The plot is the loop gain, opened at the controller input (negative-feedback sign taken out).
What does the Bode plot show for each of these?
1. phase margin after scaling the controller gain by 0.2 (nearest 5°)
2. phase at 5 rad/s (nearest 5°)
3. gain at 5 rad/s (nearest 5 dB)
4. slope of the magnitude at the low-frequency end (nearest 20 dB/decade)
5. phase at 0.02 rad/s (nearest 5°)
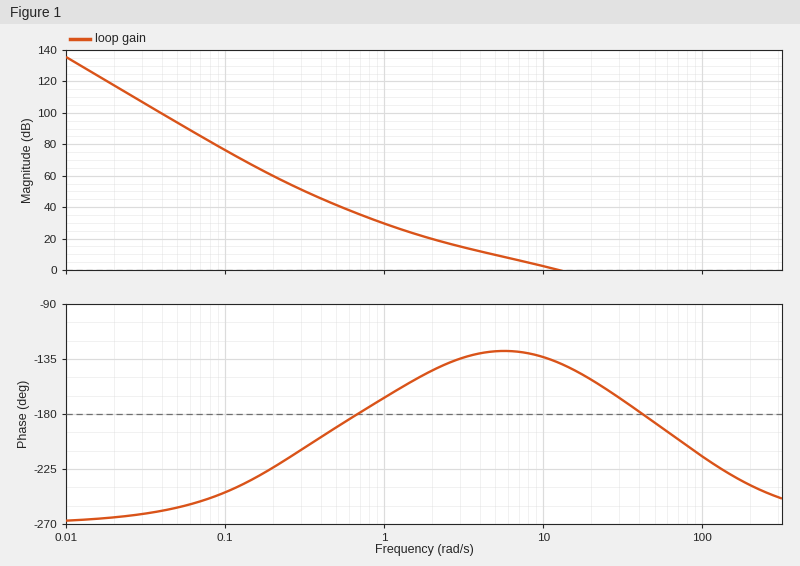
45°
-130°
10 dB
-60 dB/decade
-265°
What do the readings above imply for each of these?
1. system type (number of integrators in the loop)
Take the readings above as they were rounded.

3
